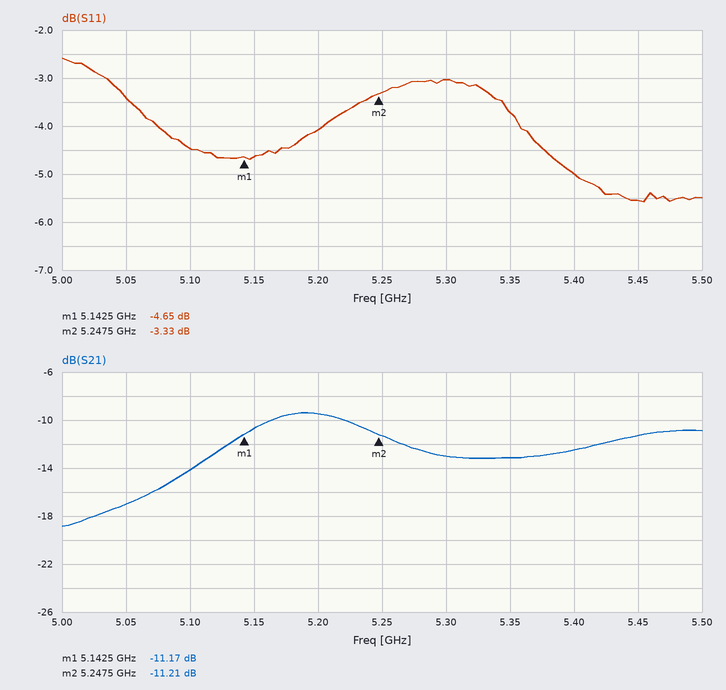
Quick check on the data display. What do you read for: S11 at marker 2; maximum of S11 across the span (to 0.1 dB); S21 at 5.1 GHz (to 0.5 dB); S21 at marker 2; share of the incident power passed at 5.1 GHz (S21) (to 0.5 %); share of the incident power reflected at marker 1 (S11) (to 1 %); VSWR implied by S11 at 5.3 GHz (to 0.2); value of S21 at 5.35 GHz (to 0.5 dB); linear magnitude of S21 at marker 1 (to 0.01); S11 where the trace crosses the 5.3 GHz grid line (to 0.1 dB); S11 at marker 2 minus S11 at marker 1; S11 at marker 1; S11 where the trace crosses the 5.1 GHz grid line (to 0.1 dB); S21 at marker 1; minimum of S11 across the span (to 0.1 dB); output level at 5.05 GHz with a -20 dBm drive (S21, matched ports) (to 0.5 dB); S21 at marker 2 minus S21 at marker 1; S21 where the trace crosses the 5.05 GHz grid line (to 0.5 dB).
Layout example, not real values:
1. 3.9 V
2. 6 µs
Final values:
1. -3.33 dB
2. -2.6 dB
3. -14.0 dB
4. -11.21 dB
5. 4.0 %
6. 34 %
7. 5.8
8. -13.0 dB
9. 0.28
10. -3.0 dB
11. 1.32 dB
12. -4.65 dB
13. -4.5 dB
14. -11.17 dB
15. -5.6 dB
16. -37.0 dBm
17. -0.04 dB
18. -17.0 dB
